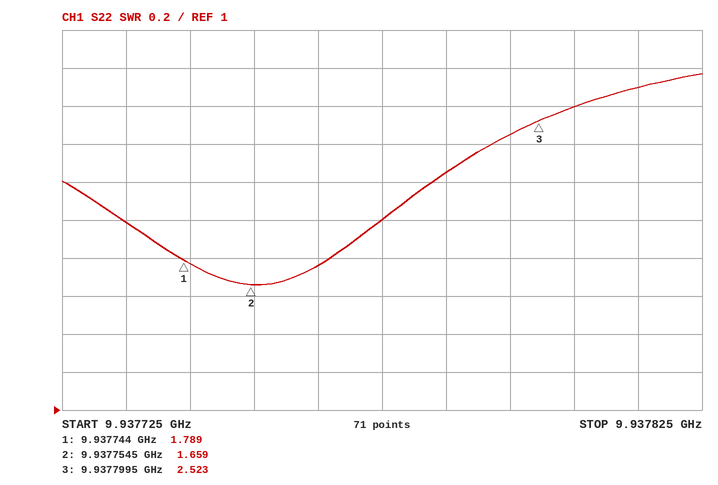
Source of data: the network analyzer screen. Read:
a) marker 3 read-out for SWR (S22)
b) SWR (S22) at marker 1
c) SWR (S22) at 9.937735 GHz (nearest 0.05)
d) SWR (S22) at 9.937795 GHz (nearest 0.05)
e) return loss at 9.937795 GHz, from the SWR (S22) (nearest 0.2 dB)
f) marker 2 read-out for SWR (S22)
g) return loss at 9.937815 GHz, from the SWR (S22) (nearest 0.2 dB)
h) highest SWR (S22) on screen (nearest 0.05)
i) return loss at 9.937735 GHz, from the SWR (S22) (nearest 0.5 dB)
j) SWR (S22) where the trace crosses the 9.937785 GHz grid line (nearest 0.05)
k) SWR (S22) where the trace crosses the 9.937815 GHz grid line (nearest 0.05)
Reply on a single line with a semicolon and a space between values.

2.523; 1.789; 2.00; 2.45; 7.6 dB; 1.659; 6.8 dB; 2.75; 9.5 dB; 2.25; 2.70
